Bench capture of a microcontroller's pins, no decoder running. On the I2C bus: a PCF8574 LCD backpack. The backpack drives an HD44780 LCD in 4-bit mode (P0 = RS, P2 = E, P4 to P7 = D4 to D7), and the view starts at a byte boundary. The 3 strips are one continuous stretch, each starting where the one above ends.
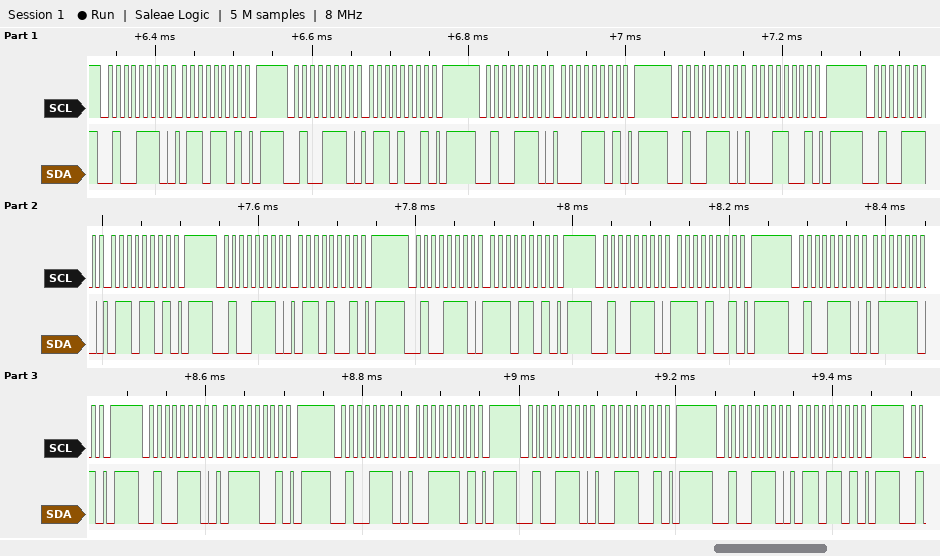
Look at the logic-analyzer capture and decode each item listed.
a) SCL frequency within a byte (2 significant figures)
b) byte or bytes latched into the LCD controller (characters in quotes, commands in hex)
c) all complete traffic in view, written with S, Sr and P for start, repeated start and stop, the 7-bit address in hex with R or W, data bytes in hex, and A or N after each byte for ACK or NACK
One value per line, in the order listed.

100 kHz
'a' 'n' 's'
S 27W A 6D A P S 27W A 69 A P S 27W A 1D A P S 27W A 19 A P S 27W A 6D A P S 27W A 69 A P S 27W A ED A P S 27W A E9 A P S 27W A 7D A P S 27W A 79 A P S 27W A 3D A P S 27W A 39 A P S 27W A 6D A P
